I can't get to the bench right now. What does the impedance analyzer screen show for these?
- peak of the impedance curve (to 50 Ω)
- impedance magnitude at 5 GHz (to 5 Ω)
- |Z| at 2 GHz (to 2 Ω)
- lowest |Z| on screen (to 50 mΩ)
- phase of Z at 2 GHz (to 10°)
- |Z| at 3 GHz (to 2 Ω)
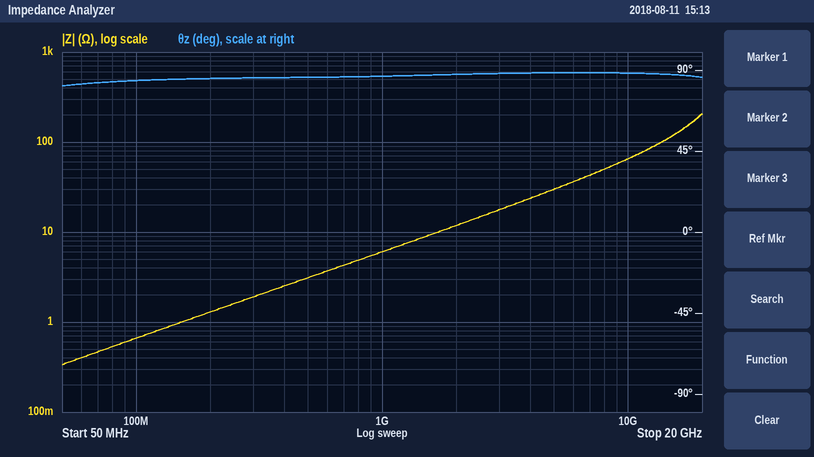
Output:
200 Ω
30 Ω
12 Ω
350 mΩ
90°
18 Ω
